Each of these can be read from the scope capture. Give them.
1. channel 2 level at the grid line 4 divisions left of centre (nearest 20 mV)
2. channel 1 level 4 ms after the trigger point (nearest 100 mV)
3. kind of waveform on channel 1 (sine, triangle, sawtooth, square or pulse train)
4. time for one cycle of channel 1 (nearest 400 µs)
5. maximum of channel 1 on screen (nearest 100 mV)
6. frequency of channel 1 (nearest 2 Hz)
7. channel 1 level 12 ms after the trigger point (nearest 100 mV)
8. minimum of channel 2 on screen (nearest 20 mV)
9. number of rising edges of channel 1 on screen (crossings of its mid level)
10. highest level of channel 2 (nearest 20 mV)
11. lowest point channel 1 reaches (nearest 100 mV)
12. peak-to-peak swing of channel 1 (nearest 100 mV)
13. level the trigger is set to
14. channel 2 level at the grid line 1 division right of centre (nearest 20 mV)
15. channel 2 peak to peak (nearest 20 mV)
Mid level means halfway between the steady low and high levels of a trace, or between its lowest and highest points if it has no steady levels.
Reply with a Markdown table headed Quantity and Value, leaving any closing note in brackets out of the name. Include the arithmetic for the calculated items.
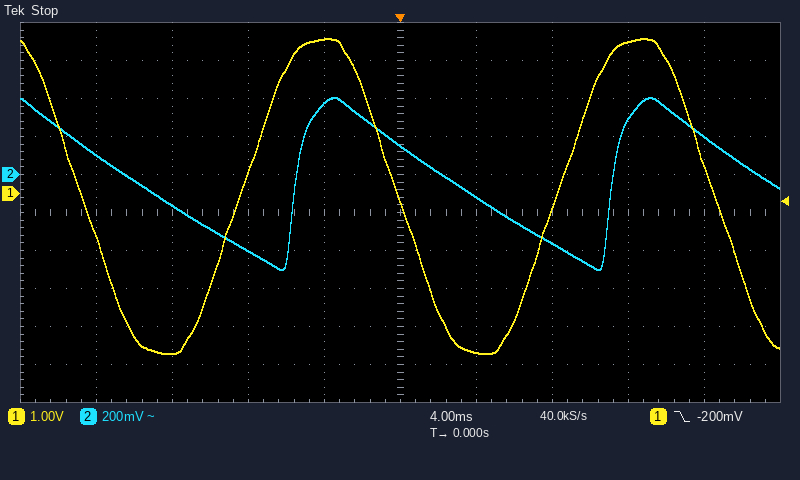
| Quantity | Value |
|---|---|
| channel 2 level at the grid line 4 divisions left of centre | 100 mV |
| channel 1 level 4 ms after the trigger point | -4.2 V |
| kind of waveform on channel 1 | sine |
| time for one cycle of channel 1 | 16.8 ms |
| maximum of channel 1 on screen | 4.1 V |
| frequency of channel 1 | 1 / 16.8 ms ≈ 60 Hz |
| channel 1 level 12 ms after the trigger point | 4.0 V |
| minimum of channel 2 on screen | -500 mV |
| number of rising edges of channel 1 on screen | 2 |
| highest level of channel 2 | 400 mV |
| lowest point channel 1 reaches | -4.2 V |
| peak-to-peak swing of channel 1 | 4.1 V − (-4.2 V) = 8.3 V |
| level the trigger is set to | -200 mV |
| channel 2 level at the grid line 1 division right of centre | -120 mV |
| channel 2 peak to peak | 400 mV − (-500 mV) = 900 mV |
